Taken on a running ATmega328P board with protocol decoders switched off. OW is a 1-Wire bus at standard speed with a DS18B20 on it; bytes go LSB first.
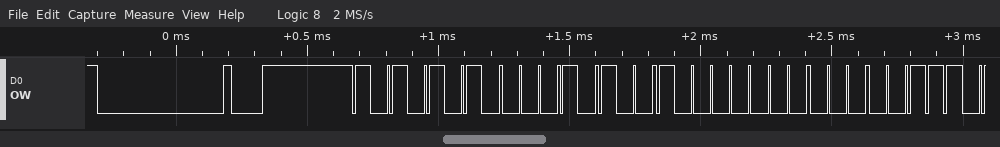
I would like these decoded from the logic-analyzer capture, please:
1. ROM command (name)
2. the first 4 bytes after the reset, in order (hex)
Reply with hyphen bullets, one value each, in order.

- Match ROM
- 55 28 01 E0
